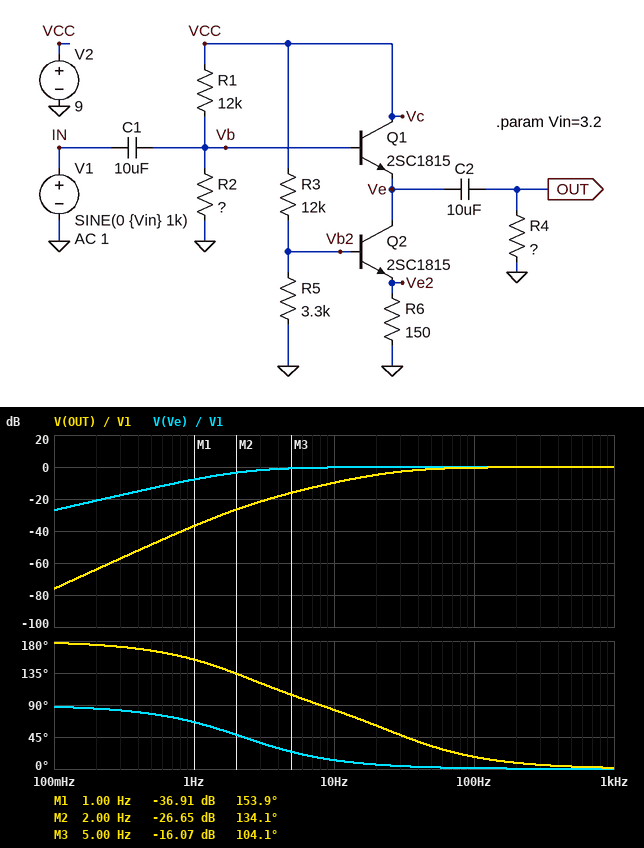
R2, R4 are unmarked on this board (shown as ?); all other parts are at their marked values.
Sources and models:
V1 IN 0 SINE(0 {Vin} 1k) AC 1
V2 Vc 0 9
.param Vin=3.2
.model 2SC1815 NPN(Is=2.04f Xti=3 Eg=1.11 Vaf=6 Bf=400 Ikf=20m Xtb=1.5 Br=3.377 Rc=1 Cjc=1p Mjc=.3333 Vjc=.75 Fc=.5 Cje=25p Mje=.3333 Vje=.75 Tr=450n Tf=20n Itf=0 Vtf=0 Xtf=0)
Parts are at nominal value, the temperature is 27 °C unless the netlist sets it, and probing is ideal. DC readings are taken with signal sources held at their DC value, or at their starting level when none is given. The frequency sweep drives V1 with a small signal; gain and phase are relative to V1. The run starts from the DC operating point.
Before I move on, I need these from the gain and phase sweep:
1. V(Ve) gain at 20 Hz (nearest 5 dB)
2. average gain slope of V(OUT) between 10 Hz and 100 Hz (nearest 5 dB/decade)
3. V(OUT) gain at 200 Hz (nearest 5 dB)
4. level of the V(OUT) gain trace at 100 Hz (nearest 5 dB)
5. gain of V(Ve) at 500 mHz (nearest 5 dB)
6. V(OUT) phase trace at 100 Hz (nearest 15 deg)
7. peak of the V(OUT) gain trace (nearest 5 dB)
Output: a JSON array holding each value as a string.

["0 dB", "10 dB/decade", "0 dB", "0 dB", "-15 dB", "15 deg", "0 dB"]
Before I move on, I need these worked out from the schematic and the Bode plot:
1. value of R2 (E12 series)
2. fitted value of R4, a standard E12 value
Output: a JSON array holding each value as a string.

["18 kΩ", "560 Ω"]
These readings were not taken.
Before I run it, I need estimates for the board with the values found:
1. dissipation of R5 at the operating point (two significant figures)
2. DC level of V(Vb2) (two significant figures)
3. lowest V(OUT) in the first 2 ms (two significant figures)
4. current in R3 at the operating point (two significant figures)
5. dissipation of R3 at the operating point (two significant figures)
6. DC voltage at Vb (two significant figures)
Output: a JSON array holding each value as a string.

["1.1 mW", "1.9 V", "-3.2 V", "590 µA", "4.2 mW", "5.3 V"]
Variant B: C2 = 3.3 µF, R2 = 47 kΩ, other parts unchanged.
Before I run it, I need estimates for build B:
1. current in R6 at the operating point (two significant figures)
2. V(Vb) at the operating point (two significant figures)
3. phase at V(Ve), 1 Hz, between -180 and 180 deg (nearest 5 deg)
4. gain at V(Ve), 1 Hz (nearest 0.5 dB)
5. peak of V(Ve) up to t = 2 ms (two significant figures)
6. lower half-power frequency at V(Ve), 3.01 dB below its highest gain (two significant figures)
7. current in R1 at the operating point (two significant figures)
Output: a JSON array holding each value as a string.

["7.8 mA", "7.0 V", "60 deg", "-6.0 dB", "9.0 V", "1.7 Hz", "170 µA"]
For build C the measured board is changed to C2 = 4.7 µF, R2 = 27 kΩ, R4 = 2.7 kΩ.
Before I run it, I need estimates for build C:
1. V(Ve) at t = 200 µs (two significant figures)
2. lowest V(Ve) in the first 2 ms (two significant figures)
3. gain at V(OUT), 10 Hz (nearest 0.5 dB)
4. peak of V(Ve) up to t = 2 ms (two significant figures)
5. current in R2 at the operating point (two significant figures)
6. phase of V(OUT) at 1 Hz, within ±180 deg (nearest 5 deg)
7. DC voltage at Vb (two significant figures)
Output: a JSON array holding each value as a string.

["8.4 V", "2.2 V", "-4.5 dB", "8.5 V", "230 µA", "150 deg", "6.1 V"]
